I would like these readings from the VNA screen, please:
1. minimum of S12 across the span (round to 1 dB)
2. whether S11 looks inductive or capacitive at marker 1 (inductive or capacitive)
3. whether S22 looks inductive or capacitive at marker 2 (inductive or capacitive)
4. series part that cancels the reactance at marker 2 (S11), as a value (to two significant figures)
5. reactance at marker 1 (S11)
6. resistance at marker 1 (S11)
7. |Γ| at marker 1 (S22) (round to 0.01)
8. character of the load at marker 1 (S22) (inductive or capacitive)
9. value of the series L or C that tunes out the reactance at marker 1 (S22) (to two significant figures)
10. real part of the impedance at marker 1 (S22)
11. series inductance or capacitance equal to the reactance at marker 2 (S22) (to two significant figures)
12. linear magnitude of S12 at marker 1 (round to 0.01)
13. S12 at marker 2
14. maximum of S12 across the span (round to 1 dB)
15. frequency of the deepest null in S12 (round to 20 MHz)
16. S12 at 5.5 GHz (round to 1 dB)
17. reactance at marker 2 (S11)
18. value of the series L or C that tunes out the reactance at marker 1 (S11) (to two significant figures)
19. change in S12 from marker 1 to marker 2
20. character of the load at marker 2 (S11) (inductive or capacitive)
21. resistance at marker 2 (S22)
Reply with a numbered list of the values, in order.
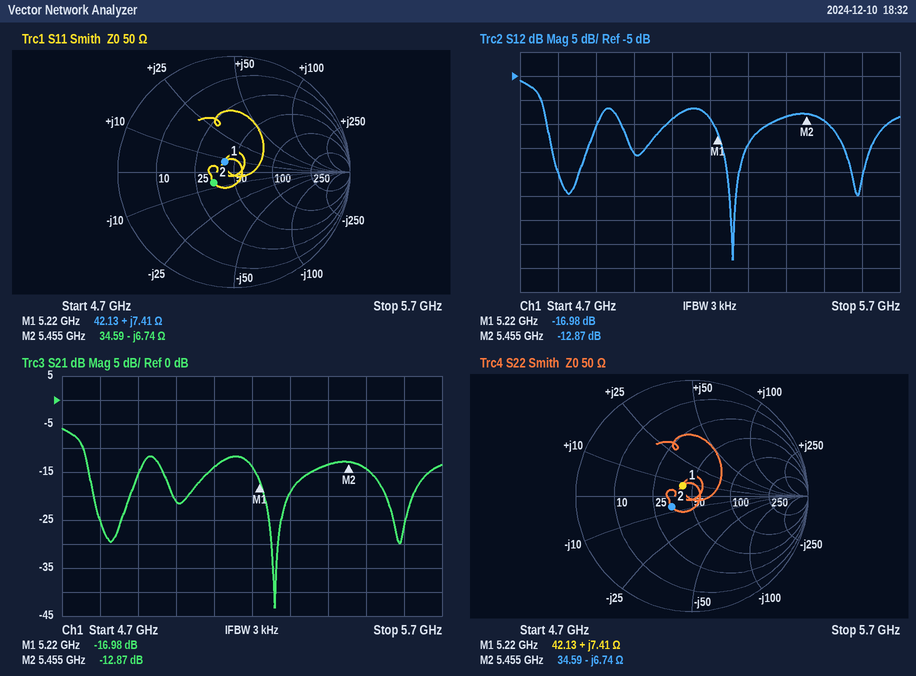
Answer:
1. -43 dB
2. inductive
3. capacitive
4. 200 pH
5. +7.41 Ω
6. 42.13 Ω
7. 0.12
8. inductive
9. 4.1 pF
10. 42.13 Ω
11. 4.3 pF
12. 0.14
13. -12.87 dB
14. -6 dB
15. 5.26 GHz
16. -14 dB
17. -6.74 Ω
18. 4.1 pF
19. 4.11 dB
20. capacitive
21. 34.59 Ω
